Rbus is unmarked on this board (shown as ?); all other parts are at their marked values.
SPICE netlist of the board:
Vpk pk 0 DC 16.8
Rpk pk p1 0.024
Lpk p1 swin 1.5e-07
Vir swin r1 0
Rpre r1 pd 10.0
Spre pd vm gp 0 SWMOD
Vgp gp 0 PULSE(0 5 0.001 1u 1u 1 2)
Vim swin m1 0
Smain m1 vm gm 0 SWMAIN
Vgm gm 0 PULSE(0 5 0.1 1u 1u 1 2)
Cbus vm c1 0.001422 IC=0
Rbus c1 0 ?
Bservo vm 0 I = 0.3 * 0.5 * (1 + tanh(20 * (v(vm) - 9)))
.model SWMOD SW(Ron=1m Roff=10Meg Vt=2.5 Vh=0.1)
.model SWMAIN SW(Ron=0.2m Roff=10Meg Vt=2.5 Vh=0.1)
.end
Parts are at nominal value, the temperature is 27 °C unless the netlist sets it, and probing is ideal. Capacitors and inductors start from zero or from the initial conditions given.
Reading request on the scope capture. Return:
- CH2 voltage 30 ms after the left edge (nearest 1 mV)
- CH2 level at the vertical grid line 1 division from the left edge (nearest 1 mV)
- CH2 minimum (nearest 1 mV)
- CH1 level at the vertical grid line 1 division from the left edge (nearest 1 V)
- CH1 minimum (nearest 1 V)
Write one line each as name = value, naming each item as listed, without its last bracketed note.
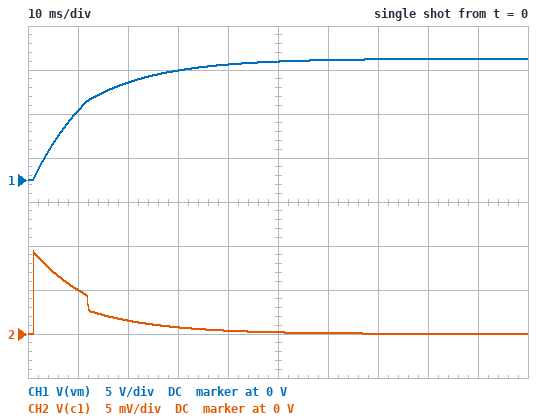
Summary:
CH2 voltage 30 ms after the left edge = 1 mV
CH2 level at the vertical grid line 1 division from the left edge = 5 mV
CH2 minimum = 0 V
CH1 level at the vertical grid line 1 division from the left edge = 8 V
CH1 minimum = 0 V
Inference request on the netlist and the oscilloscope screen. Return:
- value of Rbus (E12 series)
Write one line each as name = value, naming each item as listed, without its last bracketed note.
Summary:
value of Rbus = 5.6 mΩ
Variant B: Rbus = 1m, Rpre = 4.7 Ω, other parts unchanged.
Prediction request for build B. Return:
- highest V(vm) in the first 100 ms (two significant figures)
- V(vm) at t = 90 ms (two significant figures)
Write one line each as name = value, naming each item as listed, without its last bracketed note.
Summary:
highest V(vm) in the first 100 ms = 16 V
V(vm) at t = 90 ms = 15 V
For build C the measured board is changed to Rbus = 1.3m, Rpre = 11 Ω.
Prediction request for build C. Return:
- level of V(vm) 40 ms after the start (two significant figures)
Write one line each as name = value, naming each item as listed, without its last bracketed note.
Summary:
level of V(vm) 40 ms after the start = 13 V
